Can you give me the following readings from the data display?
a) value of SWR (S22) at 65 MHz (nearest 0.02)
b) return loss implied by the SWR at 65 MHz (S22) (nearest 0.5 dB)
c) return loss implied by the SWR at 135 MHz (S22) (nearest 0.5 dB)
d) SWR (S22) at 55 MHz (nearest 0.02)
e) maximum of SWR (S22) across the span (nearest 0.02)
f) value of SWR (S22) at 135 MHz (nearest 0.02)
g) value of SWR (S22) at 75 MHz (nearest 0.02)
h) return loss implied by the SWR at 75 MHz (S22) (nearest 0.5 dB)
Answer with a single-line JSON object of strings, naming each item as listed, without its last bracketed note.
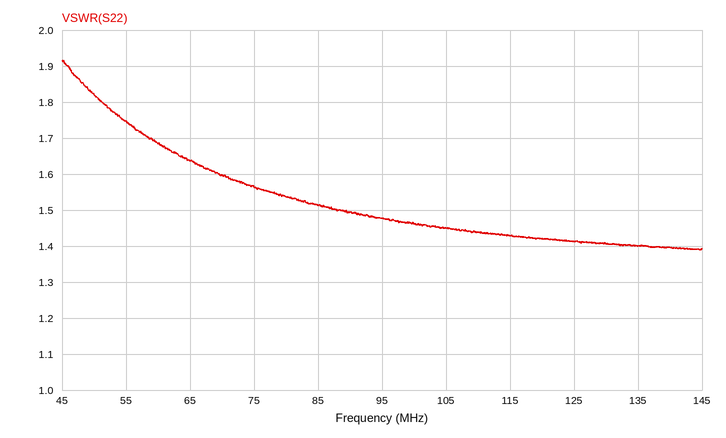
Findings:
{"value of SWR (S22) at 65 MHz": "1.64", "return loss implied by the SWR at 65 MHz (S22)": "12.5 dB", "return loss implied by the SWR at 135 MHz (S22)": "15.5 dB", "SWR (S22) at 55 MHz": "1.74", "maximum of SWR (S22) across the span": "1.92", "value of SWR (S22) at 135 MHz": "1.40", "value of SWR (S22) at 75 MHz": "1.56", "return loss implied by the SWR at 75 MHz (S22)": "13.0 dB"}
